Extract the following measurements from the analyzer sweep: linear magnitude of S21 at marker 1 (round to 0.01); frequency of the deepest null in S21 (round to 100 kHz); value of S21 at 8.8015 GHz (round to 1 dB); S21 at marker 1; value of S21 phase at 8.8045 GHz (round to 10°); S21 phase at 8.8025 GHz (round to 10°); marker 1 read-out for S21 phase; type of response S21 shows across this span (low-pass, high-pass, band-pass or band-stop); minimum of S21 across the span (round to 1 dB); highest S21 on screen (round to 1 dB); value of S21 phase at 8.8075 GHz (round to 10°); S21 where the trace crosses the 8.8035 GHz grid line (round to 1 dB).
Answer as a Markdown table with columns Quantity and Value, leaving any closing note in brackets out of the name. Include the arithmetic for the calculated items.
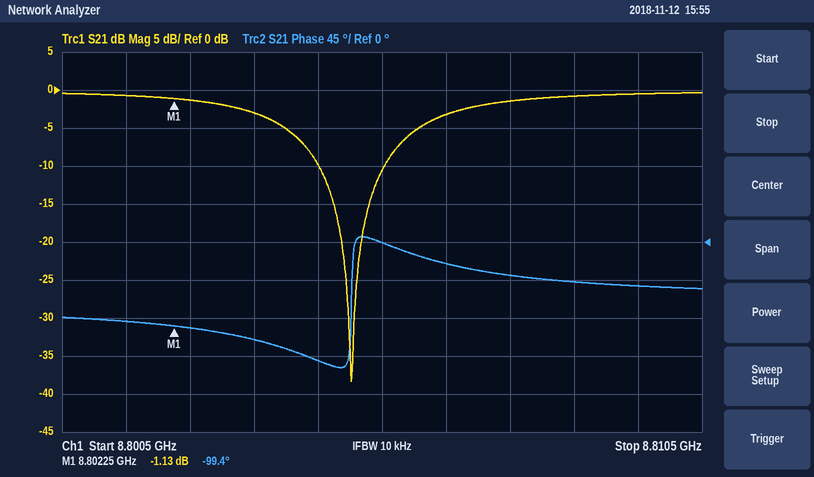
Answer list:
| Quantity | Value |
|---|---|
| linear magnitude of S21 at marker 1 | 10^(-1.13/20) ≈ 0.88 |
| frequency of the deepest null in S21 | 8.8050 GHz |
| value of S21 at 8.8015 GHz | -1 dB |
| S21 at marker 1 | -1.13 dB |
| value of S21 phase at 8.8045 GHz | -140° |
| S21 phase at 8.8025 GHz | -100° |
| marker 1 read-out for S21 phase | -99.4° |
| type of response S21 shows across this span | band-stop |
| minimum of S21 across the span | -38 dB |
| highest S21 on screen | 0 dB |
| value of S21 phase at 8.8075 GHz | -40° |
| S21 where the trace crosses the 8.8035 GHz grid line | -3 dB |
